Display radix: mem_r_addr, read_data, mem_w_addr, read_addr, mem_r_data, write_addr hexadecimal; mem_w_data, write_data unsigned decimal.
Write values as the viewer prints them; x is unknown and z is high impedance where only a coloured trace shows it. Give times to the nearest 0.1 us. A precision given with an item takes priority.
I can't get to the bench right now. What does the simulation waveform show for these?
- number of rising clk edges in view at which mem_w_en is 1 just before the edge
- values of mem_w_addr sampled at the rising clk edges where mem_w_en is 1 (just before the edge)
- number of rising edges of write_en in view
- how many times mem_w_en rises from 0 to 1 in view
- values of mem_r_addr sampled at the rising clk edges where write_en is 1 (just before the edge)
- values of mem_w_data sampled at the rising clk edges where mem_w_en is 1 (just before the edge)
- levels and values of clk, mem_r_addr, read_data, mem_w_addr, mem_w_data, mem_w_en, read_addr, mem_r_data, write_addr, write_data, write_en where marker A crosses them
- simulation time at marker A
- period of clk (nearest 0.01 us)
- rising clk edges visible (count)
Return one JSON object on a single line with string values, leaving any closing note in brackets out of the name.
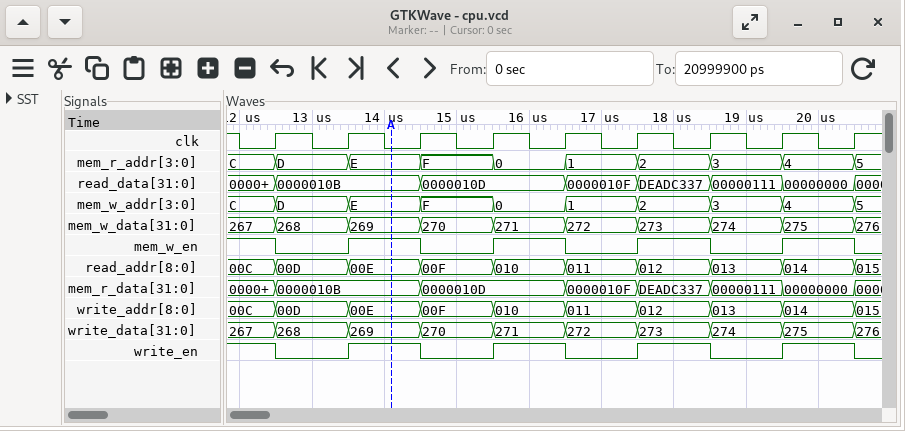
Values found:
{"number of rising clk edges in view at which mem_w_en is 1 just before the edge": "5", "values of mem_w_addr sampled at the rising clk edges where mem_w_en is 1": "C, E, 0, 2, 4", "number of rising edges of write_en in view": "4", "how many times mem_w_en rises from 0 to 1 in view": "4", "values of mem_r_addr sampled at the rising clk edges where write_en is 1": "C, E, 0, 2, 4", "values of mem_w_data sampled at the rising clk edges where mem_w_en is 1": "267, 269, 271, 273, 275", "levels and values of clk, mem_r_addr, read_data, mem_w_addr, mem_w_data, mem_w_en, read_addr, mem_r_data, write_addr, write_data, write_en where marker A crosses them": "clk=0, mem_r_addr=E, read_data=0000010B, mem_w_addr=E, mem_w_data=269, mem_w_en=1, read_addr=00E, mem_r_data=0000010B, write_addr=00E, write_data=269, write_en=1", "simulation time at marker A": "14.1 us", "period of clk": "1 us", "rising clk edges visible": "9"}
